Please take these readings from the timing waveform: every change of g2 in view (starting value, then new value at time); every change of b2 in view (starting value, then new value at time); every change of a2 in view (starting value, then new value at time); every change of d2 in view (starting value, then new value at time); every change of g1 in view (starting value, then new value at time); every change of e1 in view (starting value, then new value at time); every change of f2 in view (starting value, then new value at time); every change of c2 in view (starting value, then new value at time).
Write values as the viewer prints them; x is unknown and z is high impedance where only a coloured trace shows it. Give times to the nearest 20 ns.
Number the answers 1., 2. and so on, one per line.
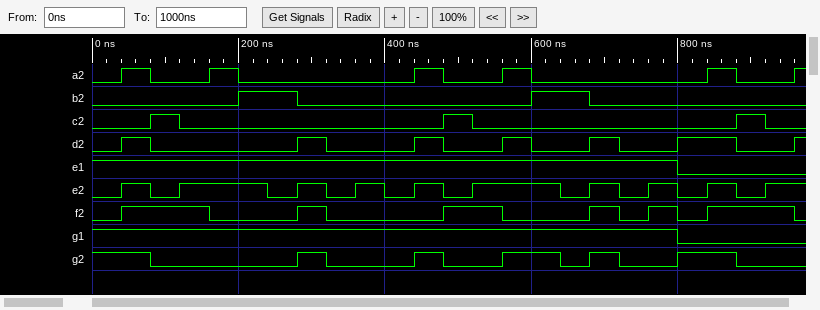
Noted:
1. 1, 0 at 80 ns, 1 at 280 ns, 0 at 320 ns, 1 at 440 ns, 0 at 480 ns, 1 at 560 ns, 0 at 640 ns, 1 at 680 ns, 0 at 720 ns, 1 at 800 ns, 0 at 880 ns
2. 0, 1 at 200 ns, 0 at 280 ns, 1 at 600 ns, 0 at 680 ns
3. 0, 1 at 40 ns, 0 at 80 ns, 1 at 160 ns, 0 at 200 ns, 1 at 440 ns, 0 at 480 ns, 1 at 560 ns, 0 at 600 ns, 1 at 840 ns, 0 at 880 ns, 1 at 960 ns
4. 0, 1 at 40 ns, 0 at 80 ns, 1 at 280 ns, 0 at 320 ns, 1 at 440 ns, 0 at 480 ns, 1 at 560 ns, 0 at 600 ns, 1 at 680 ns, 0 at 720 ns, 1 at 800 ns, 0 at 880 ns, 1 at 960 ns
5. 1, 0 at 800 ns
6. 1, 0 at 800 ns
7. 0, 1 at 40 ns, 0 at 160 ns, 1 at 280 ns, 0 at 320 ns, 1 at 480 ns, 0 at 560 ns, 1 at 680 ns, 0 at 720 ns, 1 at 760 ns, 0 at 800 ns, 1 at 840 ns, 0 at 960 ns
8. 0, 1 at 80 ns, 0 at 120 ns, 1 at 480 ns, 0 at 520 ns, 1 at 880 ns, 0 at 920 ns
